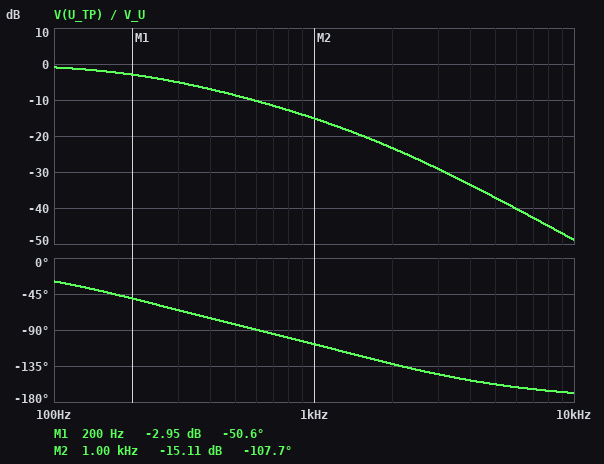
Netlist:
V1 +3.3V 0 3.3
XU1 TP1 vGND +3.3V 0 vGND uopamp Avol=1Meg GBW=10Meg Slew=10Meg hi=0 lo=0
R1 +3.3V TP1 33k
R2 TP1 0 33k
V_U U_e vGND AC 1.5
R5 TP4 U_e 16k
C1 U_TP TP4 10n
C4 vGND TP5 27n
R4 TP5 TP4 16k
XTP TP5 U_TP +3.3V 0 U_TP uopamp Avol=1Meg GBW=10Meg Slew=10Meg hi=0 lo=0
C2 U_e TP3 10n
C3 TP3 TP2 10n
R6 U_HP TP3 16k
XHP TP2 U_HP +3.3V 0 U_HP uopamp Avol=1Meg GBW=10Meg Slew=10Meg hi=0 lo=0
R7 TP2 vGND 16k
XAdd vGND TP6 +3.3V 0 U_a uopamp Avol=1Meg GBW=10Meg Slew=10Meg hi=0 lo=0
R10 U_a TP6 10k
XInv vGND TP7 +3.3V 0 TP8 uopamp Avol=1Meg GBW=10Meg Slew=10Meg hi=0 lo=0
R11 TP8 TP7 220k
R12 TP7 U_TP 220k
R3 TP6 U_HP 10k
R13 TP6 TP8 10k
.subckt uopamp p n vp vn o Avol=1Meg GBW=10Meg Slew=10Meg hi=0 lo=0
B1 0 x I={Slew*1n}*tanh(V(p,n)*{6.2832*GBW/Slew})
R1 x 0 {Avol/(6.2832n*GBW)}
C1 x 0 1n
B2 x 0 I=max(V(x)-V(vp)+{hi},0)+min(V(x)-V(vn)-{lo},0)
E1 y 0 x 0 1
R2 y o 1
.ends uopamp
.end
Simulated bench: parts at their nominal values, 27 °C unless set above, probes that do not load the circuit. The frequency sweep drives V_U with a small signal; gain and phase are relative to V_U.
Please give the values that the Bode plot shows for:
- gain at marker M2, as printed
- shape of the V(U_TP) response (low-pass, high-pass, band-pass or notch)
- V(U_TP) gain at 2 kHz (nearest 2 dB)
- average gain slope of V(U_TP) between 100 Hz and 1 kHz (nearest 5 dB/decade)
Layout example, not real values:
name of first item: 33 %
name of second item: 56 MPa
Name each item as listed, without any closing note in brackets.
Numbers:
gain at marker M2, as printed: -15.11 dB
shape of the V(U_TP) response: low-pass
V(U_TP) gain at 2 kHz: -24 dB
average gain slope of V(U_TP) between 100 Hz and 1 kHz: -15 dB/decade
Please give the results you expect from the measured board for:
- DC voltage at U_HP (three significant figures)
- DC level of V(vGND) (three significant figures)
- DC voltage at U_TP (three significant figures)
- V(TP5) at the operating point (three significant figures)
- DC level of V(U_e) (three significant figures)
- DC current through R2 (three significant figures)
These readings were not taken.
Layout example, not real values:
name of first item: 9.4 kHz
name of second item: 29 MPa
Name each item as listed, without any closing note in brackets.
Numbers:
DC voltage at U_HP: 1.65 V
DC level of V(vGND): 1.65 V
DC voltage at U_TP: 1.65 V
V(TP5) at the operating point: 1.65 V
DC level of V(U_e): 1.65 V
DC current through R2: 50.0 µA
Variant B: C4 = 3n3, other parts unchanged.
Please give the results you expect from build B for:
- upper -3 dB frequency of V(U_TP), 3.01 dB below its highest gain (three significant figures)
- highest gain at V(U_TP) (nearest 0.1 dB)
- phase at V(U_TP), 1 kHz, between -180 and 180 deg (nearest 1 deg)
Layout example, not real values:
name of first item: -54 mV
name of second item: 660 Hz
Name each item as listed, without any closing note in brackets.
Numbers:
upper -3 dB frequency of V(U_TP), 3.01 dB below its highest gain: 1.96 kHz
highest gain at V(U_TP): 0.5 dB
phase at V(U_TP), 1 kHz, between -180 and 180 deg: -45 deg
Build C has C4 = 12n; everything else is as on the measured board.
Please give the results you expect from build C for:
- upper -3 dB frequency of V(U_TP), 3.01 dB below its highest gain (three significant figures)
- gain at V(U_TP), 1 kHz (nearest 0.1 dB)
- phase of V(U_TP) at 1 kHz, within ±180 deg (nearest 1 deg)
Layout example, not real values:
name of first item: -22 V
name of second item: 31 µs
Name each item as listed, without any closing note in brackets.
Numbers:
upper -3 dB frequency of V(U_TP), 3.01 dB below its highest gain: 514 Hz
gain at V(U_TP), 1 kHz: -7.7 dB
phase of V(U_TP) at 1 kHz, within ±180 deg: -95 deg
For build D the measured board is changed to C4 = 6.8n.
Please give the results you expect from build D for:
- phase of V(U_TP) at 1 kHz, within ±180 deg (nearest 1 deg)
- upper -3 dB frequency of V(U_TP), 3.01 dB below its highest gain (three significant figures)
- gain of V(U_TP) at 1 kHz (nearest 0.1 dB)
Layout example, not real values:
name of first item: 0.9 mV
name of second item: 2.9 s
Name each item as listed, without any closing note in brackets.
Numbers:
phase of V(U_TP) at 1 kHz, within ±180 deg: -77 deg
upper -3 dB frequency of V(U_TP), 3.01 dB below its highest gain: 1.01 kHz
gain of V(U_TP) at 1 kHz: -2.9 dB
